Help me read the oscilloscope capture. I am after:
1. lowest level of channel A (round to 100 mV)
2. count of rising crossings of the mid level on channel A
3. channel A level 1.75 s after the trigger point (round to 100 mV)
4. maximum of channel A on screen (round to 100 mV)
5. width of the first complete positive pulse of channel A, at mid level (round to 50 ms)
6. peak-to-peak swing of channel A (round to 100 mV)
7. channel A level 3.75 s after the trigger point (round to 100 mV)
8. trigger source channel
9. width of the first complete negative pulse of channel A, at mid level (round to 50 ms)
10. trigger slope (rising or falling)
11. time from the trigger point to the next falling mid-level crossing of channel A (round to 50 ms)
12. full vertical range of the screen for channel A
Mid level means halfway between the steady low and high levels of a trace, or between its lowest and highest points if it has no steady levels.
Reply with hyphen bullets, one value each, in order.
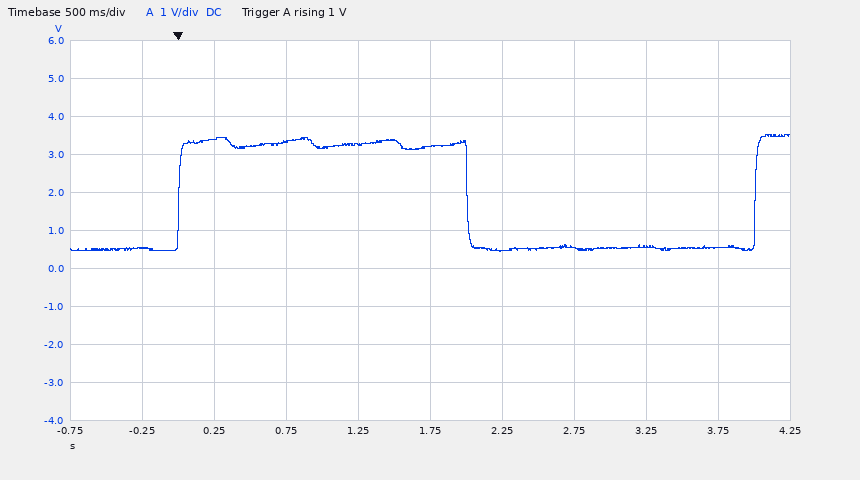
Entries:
- 400 mV
- 2
- 3.2 V
- 3.5 V
- 2.00 s
- 3.1 V
- 600 mV
- channel A
- 2.00 s
- rising
- 2.00 s
- 10 V
